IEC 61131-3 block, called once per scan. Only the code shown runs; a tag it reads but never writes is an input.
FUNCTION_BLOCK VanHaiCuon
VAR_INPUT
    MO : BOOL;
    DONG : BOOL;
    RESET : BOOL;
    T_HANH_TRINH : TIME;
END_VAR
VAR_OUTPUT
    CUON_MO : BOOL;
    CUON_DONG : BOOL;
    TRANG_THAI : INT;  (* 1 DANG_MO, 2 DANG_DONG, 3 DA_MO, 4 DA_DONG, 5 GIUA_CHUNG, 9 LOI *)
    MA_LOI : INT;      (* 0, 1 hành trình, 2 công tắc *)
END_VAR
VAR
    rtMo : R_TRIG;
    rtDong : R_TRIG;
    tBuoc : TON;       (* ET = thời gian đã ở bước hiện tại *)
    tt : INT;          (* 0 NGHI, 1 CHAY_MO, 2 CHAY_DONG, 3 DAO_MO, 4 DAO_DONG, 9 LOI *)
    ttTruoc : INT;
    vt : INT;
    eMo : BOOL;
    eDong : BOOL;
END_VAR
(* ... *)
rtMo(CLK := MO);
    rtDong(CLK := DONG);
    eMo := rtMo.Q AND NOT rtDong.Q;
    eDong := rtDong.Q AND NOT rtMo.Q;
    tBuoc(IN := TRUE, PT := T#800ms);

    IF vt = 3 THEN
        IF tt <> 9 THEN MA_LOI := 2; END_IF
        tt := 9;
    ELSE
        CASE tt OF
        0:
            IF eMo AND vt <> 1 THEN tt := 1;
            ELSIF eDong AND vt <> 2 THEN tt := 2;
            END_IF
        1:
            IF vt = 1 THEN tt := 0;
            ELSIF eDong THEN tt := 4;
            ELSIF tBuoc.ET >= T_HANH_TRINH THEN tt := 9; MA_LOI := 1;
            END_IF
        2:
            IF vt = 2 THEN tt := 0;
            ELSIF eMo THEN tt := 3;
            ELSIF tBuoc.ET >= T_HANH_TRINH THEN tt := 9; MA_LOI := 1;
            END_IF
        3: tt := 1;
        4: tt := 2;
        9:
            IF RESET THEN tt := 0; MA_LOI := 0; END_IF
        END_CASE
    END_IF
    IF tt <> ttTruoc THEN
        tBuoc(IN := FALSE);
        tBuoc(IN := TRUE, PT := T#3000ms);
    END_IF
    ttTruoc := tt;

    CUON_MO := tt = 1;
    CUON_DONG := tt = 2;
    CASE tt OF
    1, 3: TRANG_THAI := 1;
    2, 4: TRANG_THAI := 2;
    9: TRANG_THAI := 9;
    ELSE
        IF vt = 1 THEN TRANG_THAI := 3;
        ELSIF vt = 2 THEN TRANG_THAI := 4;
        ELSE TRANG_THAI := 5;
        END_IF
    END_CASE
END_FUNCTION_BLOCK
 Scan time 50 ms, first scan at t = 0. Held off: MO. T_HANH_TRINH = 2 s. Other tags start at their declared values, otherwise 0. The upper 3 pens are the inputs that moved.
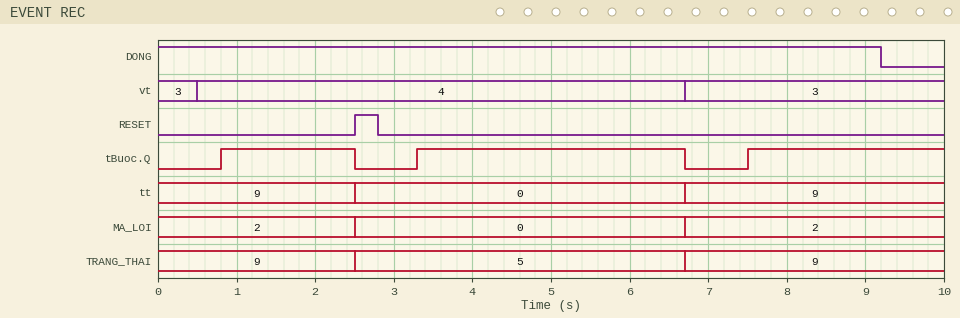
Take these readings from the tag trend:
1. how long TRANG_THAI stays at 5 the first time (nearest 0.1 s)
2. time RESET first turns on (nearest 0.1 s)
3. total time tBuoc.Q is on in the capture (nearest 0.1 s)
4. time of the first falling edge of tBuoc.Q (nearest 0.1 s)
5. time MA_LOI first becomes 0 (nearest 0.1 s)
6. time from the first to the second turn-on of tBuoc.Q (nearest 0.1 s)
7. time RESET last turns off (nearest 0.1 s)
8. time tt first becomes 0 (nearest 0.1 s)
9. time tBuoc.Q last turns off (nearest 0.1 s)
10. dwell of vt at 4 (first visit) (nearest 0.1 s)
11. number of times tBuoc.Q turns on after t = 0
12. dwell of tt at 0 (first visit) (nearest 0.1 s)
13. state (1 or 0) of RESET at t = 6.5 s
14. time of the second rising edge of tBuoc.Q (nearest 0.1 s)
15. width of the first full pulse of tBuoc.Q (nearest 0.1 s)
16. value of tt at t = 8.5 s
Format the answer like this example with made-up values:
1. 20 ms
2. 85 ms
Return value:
1. 4.2 s
2. 2.5 s
3. 7.6 s
4. 2.5 s
5. 2.5 s
6. 2.5 s
7. 2.8 s
8. 2.5 s
9. 6.7 s
10. 6.2 s
11. 3
12. 4.2 s
13. 0
14. 3.3 s
15. 1.7 s
16. 9
